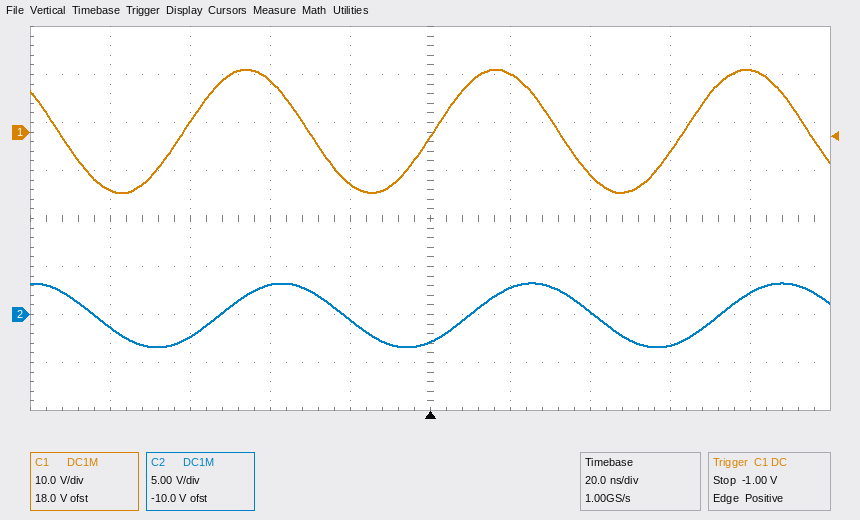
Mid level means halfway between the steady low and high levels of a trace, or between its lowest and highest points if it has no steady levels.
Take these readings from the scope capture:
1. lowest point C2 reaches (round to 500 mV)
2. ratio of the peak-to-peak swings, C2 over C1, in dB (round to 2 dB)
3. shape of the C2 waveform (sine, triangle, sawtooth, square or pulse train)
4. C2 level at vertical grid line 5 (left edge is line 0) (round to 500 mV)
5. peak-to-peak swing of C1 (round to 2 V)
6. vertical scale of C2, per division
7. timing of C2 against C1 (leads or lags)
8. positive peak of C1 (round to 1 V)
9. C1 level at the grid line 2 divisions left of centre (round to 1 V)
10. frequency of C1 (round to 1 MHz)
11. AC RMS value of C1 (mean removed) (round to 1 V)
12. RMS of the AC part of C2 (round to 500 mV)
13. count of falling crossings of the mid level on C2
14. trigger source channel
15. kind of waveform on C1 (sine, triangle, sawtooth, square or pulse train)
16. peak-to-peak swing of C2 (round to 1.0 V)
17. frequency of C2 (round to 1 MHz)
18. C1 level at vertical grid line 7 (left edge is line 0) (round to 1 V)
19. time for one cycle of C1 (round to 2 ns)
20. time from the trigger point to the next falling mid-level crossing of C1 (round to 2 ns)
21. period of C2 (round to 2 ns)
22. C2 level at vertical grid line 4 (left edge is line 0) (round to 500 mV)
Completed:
-3.5 V
-12 dB
sine
-3.0 V
26 V
5 V
lags
13 V
11 V
16 MHz
9 V
2.5 V
3
C1
sine
7.0 V
16 MHz
-9 V
62 ns
32 ns
62 ns
-500 mV
